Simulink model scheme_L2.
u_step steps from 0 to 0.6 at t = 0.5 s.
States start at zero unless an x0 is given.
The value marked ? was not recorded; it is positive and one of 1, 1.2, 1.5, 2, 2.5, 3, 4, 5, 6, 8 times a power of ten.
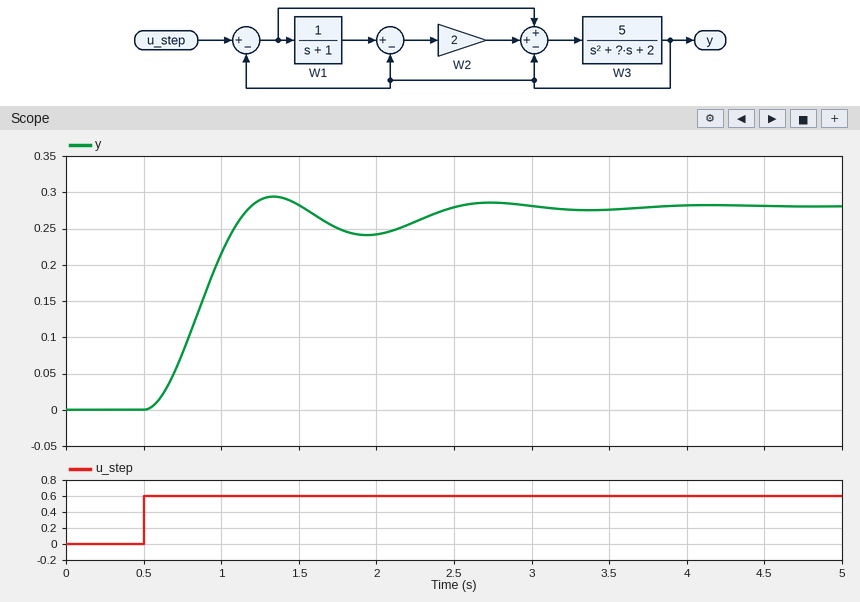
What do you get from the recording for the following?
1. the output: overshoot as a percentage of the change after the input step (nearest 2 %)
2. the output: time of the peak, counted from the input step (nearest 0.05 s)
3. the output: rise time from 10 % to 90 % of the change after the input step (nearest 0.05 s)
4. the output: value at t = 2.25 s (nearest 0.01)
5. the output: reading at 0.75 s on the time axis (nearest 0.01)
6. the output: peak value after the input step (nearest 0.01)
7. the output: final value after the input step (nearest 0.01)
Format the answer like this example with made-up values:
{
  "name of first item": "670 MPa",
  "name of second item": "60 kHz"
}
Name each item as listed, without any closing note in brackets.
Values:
{
  "the output: overshoot as a percentage of the change after the input step": "4 %",
  "the output: time of the peak, counted from the input step": "0.85 s",
  "the output: rise time from 10 % to 90 % of the change after the input step": "0.45 s",
  "the output: value at t = 2.25 s": "0.26",
  "the output: reading at 0.75 s on the time axis": "0.08",
  "the output: peak value after the input step": "0.29",
  "the output: final value after the input step": "0.28"
}
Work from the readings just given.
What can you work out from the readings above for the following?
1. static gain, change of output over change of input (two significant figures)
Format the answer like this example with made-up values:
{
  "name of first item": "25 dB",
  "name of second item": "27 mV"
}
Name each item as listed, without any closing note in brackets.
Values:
{
  "static gain, change of output over change of input": "0.47"
}
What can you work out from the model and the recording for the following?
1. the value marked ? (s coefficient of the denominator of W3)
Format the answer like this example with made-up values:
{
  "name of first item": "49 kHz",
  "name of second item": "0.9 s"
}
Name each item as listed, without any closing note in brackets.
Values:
{
  "the value marked ?": "3"
}
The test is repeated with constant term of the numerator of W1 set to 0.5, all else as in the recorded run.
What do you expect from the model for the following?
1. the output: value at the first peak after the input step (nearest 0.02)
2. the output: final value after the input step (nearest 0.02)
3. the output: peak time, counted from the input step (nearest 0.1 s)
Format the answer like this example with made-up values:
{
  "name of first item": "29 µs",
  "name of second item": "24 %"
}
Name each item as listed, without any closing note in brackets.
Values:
{
  "the output: value at the first peak after the input step": "0.24",
  "the output: final value after the input step": "0.22",
  "the output: peak time, counted from the input step": "0.8 s"
}
